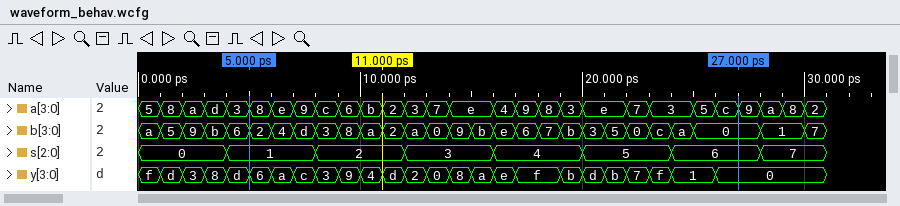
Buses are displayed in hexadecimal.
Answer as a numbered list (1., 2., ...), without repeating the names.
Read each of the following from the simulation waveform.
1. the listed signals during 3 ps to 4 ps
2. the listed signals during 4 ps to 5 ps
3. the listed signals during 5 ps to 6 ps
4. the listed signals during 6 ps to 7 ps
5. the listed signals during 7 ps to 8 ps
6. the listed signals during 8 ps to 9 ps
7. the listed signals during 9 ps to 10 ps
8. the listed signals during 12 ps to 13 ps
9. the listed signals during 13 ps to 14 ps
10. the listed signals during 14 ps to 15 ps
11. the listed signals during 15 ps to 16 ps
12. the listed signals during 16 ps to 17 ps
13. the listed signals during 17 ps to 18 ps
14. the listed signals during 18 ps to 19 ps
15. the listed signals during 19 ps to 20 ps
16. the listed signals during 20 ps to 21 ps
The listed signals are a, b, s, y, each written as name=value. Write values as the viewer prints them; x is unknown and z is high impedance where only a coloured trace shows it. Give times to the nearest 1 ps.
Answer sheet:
1. a=d, b=b, s=0, y=8
2. a=3, b=6, s=1, y=d
3. a=8, b=2, s=1, y=6
4. a=e, b=4, s=1, y=a
5. a=9, b=d, s=1, y=c
6. a=c, b=3, s=2, y=3
7. a=6, b=8, s=2, y=9
8. a=3, b=a, s=3, y=2
9. a=7, b=0, s=3, y=0
10. a=e, b=9, s=3, y=8
11. a=e, b=b, s=3, y=a
12. a=4, b=e, s=4, y=e
13. a=9, b=6, s=4, y=f
14. a=8, b=7, s=4, y=f
15. a=3, b=b, s=4, y=b
16. a=e, b=3, s=5, y=d
